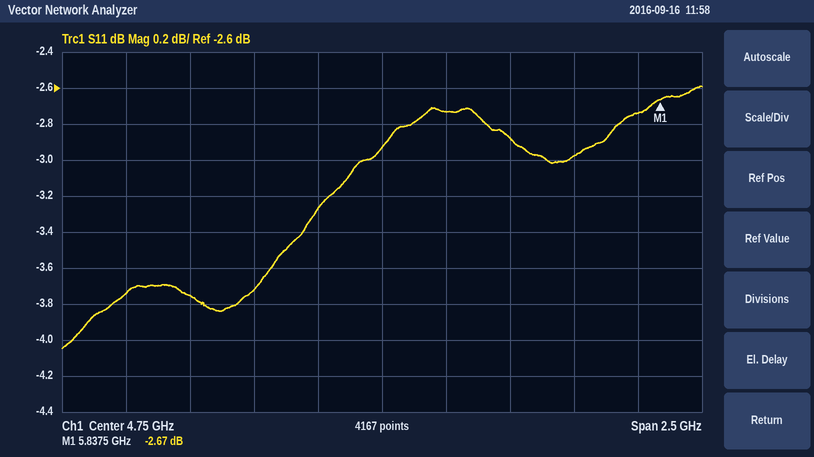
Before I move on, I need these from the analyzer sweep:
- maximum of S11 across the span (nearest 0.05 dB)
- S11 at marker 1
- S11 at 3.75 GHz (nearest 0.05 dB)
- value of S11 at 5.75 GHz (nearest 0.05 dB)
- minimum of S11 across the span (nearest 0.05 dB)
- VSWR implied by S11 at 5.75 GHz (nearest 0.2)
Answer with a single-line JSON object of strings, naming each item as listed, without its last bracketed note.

{"maximum of S11 across the span": "-2.60 dB", "S11 at marker 1": "-2.67 dB", "S11 at 3.75 GHz": "-3.75 dB", "value of S11 at 5.75 GHz": "-2.75 dB", "minimum of S11 across the span": "-4.05 dB", "VSWR implied by S11 at 5.75 GHz": "6.4"}
